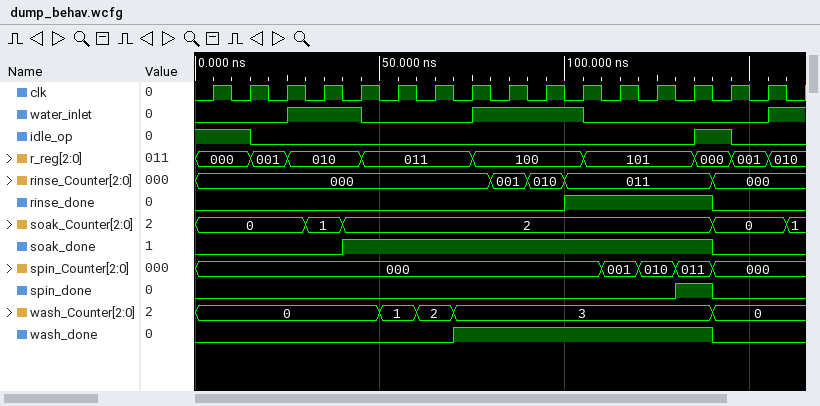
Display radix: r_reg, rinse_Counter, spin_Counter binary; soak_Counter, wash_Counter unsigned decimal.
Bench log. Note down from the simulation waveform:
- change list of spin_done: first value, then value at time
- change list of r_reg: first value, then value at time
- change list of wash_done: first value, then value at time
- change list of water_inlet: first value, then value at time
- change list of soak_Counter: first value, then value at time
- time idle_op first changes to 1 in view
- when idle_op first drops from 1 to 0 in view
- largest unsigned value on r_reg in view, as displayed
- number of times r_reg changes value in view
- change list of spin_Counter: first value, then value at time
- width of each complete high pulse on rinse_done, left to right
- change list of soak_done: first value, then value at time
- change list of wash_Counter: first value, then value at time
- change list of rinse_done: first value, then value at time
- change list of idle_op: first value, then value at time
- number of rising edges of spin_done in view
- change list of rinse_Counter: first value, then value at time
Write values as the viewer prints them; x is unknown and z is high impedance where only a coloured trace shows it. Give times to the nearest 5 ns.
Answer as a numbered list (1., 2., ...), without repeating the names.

1. 0, 1 at 130 ns, 0 at 140 ns
2. 000, 001 at 15 ns, 010 at 25 ns, 011 at 45 ns, 100 at 75 ns, 101 at 105 ns, 000 at 135 ns, 001 at 145 ns, 010 at 155 ns
3. 0, 1 at 70 ns, 0 at 140 ns
4. 0, 1 at 25 ns, 0 at 45 ns, 1 at 75 ns, 0 at 105 ns, 1 at 155 ns
5. 0, 1 at 30 ns, 2 at 40 ns, 0 at 140 ns, 1 at 160 ns
6. 135 ns
7. 15 ns
8. 101
9. 8
10. 000, 001 at 110 ns, 010 at 120 ns, 011 at 130 ns, 000 at 140 ns
11. 40 ns
12. 0, 1 at 40 ns, 0 at 140 ns
13. 0, 1 at 50 ns, 2 at 60 ns, 3 at 70 ns, 0 at 140 ns
14. 0, 1 at 100 ns, 0 at 140 ns
15. 1, 0 at 15 ns, 1 at 135 ns, 0 at 145 ns
16. 1
17. 000, 001 at 80 ns, 010 at 90 ns, 011 at 100 ns, 000 at 140 ns
